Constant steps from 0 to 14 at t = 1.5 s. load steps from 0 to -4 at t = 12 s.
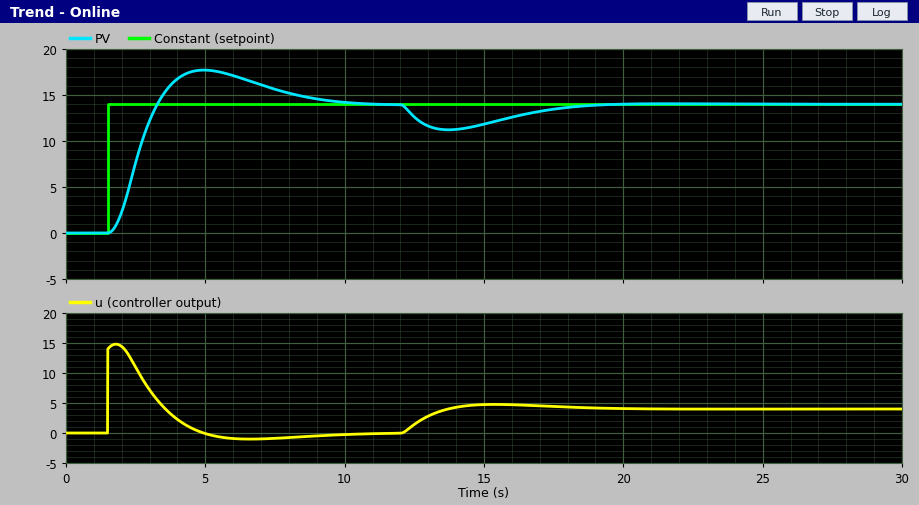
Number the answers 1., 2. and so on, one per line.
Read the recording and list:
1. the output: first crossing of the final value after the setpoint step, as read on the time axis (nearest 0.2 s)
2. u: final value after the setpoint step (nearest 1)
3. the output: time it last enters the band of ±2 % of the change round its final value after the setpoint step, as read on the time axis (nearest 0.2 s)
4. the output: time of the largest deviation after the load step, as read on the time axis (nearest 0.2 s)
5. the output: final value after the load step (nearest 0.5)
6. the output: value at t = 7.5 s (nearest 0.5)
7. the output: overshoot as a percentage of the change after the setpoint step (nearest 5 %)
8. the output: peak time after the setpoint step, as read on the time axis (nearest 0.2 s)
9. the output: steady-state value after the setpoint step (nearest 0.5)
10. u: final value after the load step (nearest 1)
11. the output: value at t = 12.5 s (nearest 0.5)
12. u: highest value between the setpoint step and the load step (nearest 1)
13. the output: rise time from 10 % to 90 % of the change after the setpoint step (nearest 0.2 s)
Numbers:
1. 3.2 s
2. 0
3. 9.8 s
4. 13.8 s
5. 14.0
6. 15.5
7. 25 %
8. 5.0 s
9. 14.0
10. 4
11. 12.5
12. 15
13. 1.2 s
